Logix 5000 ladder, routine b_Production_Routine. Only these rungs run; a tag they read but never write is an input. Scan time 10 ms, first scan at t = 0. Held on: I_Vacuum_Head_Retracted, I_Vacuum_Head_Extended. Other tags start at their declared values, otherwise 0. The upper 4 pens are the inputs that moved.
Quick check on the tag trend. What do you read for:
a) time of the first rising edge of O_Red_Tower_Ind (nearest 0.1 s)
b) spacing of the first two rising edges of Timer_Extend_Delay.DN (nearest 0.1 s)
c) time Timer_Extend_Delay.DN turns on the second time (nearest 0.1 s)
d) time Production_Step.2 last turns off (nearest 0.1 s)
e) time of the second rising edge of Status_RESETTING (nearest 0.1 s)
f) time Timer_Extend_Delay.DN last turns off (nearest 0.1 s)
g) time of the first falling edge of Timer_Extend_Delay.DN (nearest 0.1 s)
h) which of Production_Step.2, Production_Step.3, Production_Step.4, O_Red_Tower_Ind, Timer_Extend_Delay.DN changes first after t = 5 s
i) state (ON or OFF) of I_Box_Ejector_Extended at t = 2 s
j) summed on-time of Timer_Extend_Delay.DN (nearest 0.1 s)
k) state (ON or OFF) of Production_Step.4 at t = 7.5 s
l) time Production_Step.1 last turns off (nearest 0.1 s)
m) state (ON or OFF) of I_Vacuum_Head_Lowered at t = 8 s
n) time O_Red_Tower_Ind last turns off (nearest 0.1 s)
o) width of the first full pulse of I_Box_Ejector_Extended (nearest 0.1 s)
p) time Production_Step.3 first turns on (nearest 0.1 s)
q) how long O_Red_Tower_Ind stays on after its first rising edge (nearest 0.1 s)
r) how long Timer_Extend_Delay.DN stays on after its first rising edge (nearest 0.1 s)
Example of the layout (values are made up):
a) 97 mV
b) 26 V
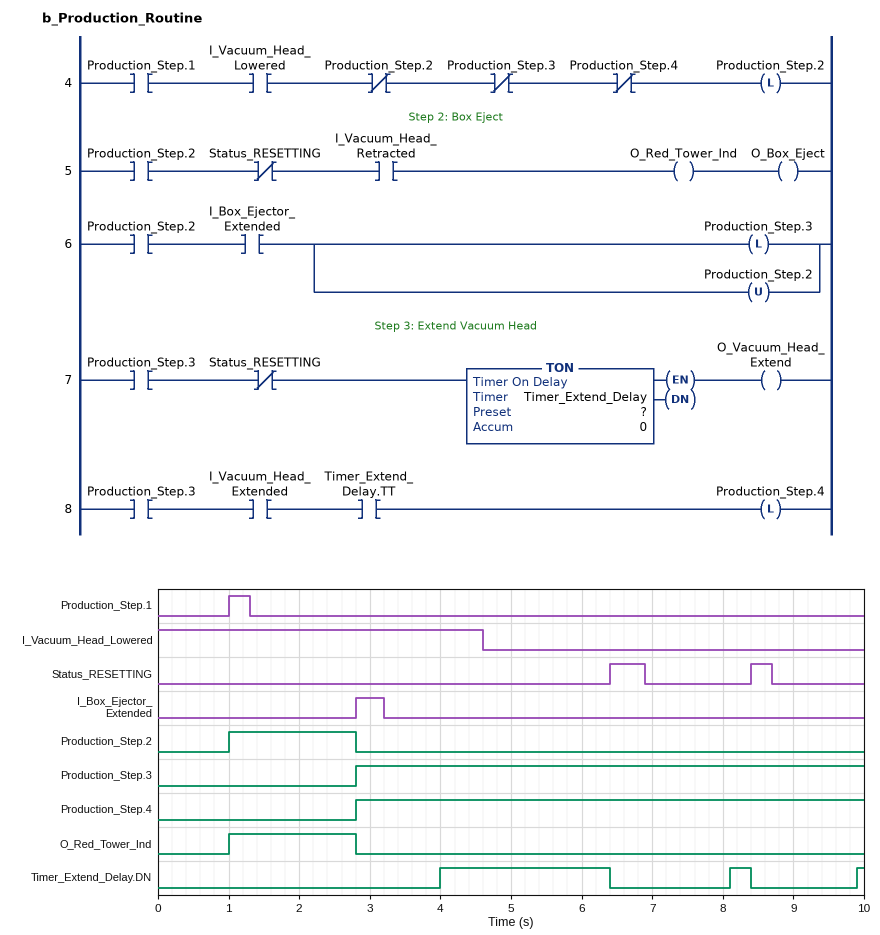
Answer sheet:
a) 1.0 s
b) 4.1 s
c) 8.1 s
d) 2.8 s
e) 8.4 s
f) 8.4 s
g) 6.4 s
h) Timer_Extend_Delay.DN
i) OFF
j) 2.8 s
k) ON
l) 1.3 s
m) OFF
n) 2.8 s
o) 0.4 s
p) 2.8 s
q) 1.8 s
r) 2.4 s
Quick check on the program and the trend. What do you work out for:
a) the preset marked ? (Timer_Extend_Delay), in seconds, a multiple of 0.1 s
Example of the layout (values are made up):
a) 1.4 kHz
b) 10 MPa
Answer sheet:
a) 1.2 s
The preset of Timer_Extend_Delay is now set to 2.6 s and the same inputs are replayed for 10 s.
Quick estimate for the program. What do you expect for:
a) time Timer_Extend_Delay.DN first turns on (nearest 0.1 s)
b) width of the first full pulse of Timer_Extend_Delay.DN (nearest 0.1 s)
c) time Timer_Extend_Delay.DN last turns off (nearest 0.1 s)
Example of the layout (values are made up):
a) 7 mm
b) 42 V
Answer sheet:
a) 5.4 s
b) 1.0 s
c) 6.4 s
